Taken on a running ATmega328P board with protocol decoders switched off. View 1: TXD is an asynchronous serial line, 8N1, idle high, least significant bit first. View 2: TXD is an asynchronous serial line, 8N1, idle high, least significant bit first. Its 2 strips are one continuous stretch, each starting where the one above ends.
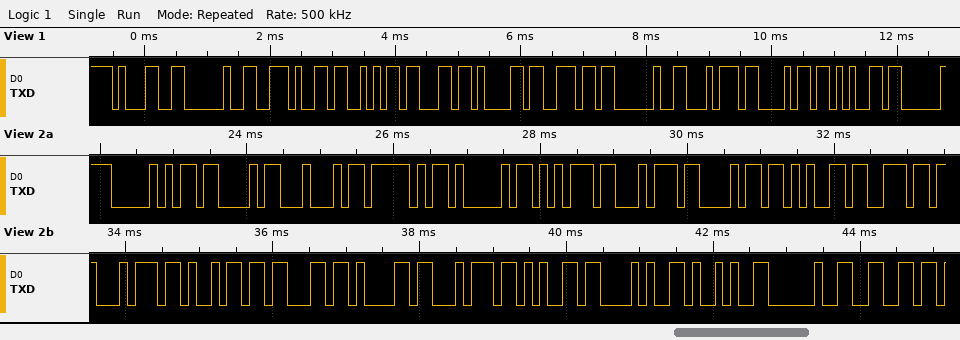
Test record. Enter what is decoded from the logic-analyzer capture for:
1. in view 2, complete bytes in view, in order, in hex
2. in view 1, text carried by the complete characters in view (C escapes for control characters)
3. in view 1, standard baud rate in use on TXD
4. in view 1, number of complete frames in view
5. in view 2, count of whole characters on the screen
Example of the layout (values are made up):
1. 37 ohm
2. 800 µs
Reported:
1. 50 43 44 5F 41 75 74 68 65 6E 74 69 63 61 74 65 28 29 20 66
2. "1 .Scan the"
3. 9600 baud
4. 11
5. 20
